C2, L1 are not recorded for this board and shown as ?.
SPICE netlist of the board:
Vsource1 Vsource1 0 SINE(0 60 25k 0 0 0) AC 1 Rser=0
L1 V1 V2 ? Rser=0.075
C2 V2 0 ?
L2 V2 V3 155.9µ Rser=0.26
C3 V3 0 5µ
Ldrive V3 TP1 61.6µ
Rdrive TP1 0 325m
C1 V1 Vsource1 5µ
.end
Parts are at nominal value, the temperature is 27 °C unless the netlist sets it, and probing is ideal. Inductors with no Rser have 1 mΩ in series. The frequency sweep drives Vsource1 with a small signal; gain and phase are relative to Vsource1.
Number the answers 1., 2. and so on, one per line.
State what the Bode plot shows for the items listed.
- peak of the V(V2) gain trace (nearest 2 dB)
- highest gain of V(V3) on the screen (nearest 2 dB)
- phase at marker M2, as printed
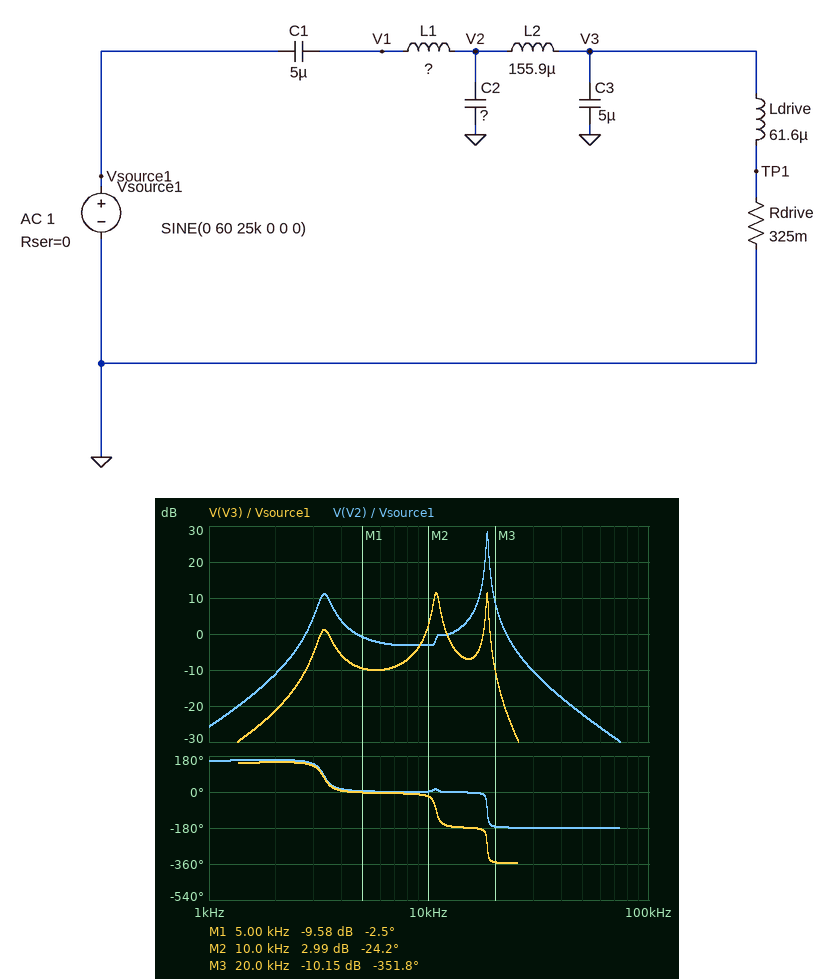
1. 28 dB
2. 12 dB
3. -24.2 deg
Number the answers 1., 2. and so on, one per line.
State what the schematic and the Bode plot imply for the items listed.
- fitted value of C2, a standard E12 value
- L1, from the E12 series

1. 4.7 µF
2. 33 µH
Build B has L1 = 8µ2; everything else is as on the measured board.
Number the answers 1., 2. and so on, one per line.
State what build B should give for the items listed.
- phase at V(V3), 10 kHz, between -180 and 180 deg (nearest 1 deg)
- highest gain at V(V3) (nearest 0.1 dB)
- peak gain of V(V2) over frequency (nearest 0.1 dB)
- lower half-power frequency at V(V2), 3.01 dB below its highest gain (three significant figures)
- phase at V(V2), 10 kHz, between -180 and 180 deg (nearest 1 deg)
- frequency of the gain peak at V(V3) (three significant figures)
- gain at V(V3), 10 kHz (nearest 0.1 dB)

1. -21 deg
2. 9.1 dB
3. 22.2 dB
4. 35.2 kHz
5. 6 deg
6. 10.9 kHz
7. -0.1 dB
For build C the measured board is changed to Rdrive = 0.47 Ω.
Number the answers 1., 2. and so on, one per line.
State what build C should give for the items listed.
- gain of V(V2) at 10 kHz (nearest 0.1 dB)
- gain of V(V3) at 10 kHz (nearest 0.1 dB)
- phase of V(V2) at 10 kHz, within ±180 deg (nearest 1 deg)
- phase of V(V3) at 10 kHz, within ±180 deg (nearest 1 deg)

1. -2.9 dB
2. 2.6 dB
3. 4 deg
4. -33 deg
